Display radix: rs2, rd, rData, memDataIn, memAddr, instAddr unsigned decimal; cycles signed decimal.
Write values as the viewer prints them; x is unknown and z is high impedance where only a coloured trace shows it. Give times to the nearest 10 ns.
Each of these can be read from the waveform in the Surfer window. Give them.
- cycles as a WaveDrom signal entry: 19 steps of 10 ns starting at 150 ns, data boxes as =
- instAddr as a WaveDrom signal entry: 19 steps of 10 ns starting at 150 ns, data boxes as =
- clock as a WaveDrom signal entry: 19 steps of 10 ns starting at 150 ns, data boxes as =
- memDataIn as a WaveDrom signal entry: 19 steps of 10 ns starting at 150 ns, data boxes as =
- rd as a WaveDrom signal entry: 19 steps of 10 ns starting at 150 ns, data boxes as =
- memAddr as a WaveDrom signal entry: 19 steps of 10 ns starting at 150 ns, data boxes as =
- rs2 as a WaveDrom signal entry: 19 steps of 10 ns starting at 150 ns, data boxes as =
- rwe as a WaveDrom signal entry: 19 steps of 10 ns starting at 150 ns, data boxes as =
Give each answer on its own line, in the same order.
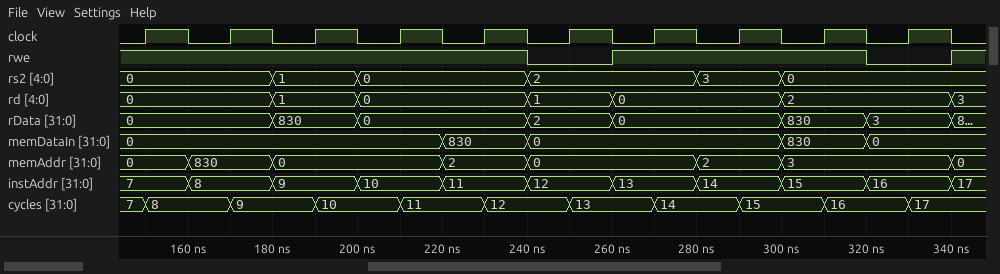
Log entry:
{name: 'cycles', wave: '=.=.=.=.=.=.=.=.=.=', data: '8 9 10 11 12 13 14 15 16 17'}
{name: 'instAddr', wave: '==.=.=.=.=.=.=.=.=.', data: '7 8 9 10 11 12 13 14 15 16'}
{name: 'clock', wave: '1010101010101010101'}
{name: 'memDataIn', wave: '=......=.=.....=.=.', data: '0 830 0 830 0'}
{name: 'rd', wave: '=..=.=...=.=...=...', data: '0 1 0 1 0 2'}
{name: 'memAddr', wave: '==.=...=.=...=.=...', data: '0 830 0 2 0 2 3'}
{name: 'rs2', wave: '=..=.=...=...=.=...', data: '0 1 0 2 3 0'}
{name: 'rwe', wave: '1........0.1.....0.'}
